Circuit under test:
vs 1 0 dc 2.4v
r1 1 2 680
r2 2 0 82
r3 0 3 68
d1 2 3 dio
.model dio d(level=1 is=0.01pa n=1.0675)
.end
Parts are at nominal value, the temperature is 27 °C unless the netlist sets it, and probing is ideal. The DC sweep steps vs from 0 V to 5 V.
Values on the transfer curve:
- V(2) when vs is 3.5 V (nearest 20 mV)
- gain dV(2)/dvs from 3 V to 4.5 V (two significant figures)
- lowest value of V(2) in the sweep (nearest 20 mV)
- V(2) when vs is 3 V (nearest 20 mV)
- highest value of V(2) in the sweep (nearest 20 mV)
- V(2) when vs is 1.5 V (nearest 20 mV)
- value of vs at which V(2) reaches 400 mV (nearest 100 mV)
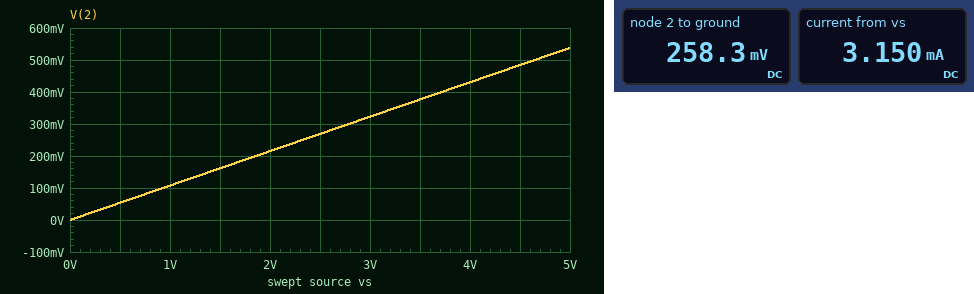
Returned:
380 mV
0.11 V/V
0 V
320 mV
540 mV
160 mV
3.7 V
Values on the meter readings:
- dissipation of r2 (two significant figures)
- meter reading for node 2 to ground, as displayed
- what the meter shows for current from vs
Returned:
810 µW
258.3 mV
3.150 mA
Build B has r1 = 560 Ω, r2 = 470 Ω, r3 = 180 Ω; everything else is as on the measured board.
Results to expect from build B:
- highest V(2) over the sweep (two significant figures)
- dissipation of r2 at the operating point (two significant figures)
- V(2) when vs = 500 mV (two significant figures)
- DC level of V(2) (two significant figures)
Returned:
1.4 V
1.6 mW
230 mV
860 mV
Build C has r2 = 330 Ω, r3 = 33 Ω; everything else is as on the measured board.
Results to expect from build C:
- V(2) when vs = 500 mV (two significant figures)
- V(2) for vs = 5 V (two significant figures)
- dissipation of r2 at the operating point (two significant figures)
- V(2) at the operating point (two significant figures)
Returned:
160 mV
850 mV
1.4 mW
690 mV
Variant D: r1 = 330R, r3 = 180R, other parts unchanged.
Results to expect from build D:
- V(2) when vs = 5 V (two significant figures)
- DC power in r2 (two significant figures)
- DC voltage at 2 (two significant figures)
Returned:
920 mV
2.8 mW
480 mV
